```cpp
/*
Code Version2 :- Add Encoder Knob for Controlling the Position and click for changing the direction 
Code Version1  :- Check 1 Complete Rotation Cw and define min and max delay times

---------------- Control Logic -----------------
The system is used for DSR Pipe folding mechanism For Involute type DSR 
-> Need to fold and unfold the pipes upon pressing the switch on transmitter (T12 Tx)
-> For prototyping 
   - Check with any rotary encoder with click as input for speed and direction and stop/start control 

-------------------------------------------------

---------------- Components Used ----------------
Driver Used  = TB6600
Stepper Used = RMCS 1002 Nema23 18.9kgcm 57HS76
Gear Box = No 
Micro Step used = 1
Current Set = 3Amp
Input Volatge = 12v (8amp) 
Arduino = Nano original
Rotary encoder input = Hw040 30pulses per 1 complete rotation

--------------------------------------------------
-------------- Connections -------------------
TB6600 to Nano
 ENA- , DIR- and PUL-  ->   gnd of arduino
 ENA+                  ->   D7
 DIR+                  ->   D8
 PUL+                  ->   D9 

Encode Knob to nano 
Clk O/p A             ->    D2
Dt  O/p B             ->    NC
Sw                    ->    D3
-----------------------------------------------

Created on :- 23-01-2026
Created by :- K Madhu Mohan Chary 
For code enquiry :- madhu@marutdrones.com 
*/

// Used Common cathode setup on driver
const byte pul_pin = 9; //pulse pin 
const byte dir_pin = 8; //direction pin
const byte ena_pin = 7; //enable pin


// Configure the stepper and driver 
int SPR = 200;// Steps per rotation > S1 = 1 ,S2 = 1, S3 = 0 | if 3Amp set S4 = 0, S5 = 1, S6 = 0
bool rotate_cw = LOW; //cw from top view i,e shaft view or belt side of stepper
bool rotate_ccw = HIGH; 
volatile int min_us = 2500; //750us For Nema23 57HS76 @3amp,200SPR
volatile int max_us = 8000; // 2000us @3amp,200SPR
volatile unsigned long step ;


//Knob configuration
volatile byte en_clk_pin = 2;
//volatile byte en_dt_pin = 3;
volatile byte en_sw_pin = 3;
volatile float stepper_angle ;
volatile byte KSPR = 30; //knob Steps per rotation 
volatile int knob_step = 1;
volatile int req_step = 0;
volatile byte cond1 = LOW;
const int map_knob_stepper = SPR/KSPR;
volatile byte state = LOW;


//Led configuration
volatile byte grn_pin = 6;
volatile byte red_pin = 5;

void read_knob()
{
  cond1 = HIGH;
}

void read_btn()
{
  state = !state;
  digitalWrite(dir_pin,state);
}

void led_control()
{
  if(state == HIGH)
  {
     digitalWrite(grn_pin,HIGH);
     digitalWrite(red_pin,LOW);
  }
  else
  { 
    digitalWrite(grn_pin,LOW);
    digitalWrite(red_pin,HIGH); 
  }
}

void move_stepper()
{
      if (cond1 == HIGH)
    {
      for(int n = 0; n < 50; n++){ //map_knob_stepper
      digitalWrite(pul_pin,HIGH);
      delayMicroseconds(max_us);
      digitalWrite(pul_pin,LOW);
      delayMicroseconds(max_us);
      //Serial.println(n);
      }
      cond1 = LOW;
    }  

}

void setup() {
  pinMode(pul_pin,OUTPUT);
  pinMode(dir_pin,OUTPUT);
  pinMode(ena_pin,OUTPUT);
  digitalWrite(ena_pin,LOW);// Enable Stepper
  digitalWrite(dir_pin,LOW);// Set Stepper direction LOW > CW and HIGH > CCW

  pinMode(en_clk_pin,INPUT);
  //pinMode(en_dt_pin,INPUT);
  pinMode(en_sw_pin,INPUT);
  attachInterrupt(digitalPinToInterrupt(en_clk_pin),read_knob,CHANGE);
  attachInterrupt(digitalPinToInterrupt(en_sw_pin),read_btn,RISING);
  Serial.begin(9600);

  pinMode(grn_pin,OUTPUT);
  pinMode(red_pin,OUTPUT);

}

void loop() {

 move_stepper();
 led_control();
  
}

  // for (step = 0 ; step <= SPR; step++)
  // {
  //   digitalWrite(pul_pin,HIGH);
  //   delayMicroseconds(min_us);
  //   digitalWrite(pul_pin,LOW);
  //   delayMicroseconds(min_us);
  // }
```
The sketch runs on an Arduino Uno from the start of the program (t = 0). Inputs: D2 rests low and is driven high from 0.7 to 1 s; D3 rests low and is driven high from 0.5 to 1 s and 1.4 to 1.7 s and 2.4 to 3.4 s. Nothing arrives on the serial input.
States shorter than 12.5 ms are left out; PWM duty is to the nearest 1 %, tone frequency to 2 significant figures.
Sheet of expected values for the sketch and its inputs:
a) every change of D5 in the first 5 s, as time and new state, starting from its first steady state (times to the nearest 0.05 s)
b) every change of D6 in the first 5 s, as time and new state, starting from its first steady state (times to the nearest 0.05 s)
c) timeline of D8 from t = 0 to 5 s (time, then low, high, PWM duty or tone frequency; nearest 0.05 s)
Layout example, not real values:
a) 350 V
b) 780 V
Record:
a) 0 s high; 0.5 s low; 1.5 s high; 2.4 s low
b) 0 s low; 0.5 s high; 1.5 s low; 2.4 s high
c) 0 s low; 0.5 s high; 1.4 s low; 2.4 s high
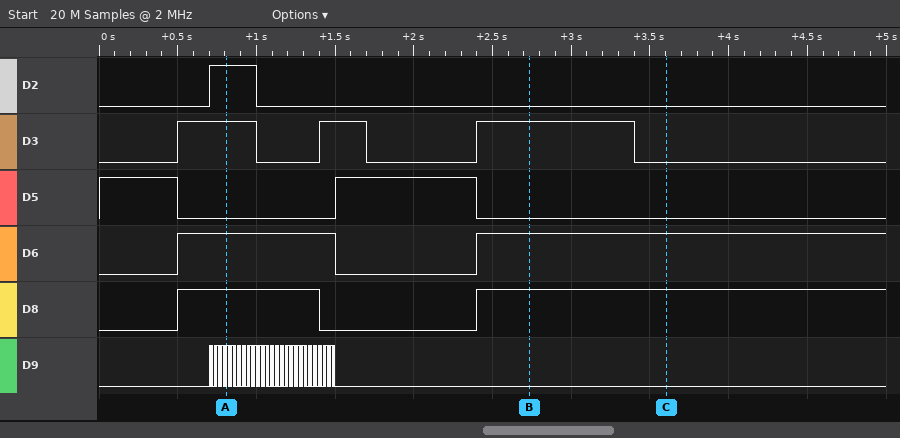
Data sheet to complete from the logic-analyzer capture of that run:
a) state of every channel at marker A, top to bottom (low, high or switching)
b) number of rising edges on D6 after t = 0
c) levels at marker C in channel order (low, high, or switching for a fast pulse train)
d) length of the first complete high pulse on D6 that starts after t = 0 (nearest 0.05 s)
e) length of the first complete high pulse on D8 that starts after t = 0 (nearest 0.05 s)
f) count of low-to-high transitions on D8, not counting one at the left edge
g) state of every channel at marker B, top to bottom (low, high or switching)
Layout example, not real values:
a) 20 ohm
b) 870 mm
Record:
a) D2 high, D3 high, D5 low, D6 high, D8 high, D9 switching
b) 2
c) D2 low, D3 low, D5 low, D6 high, D8 high, D9 low
d) 1.00 s
e) 0.90 s
f) 2
g) D2 low, D3 high, D5 low, D6 high, D8 high, D9 low
